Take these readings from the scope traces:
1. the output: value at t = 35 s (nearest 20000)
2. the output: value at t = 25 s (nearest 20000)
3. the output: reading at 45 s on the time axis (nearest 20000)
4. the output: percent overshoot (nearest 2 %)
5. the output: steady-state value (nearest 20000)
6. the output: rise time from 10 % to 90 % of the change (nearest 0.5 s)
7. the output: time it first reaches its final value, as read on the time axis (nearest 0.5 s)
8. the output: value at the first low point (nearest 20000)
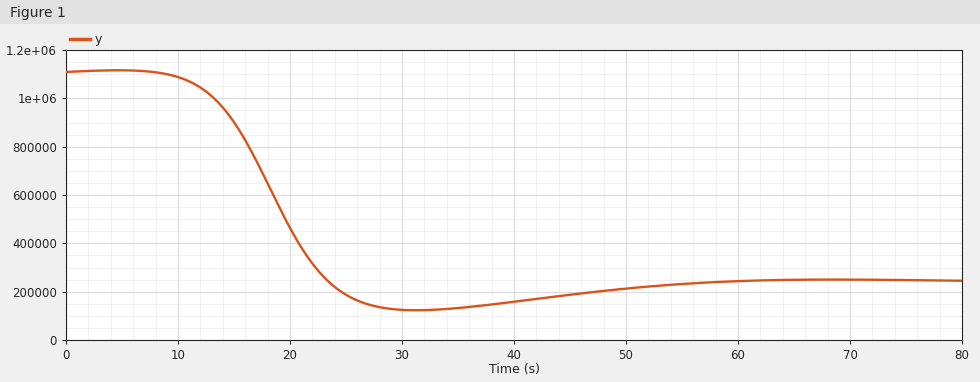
140000
180000
180000
14 %
240000
9.0 s
23.5 s
120000
